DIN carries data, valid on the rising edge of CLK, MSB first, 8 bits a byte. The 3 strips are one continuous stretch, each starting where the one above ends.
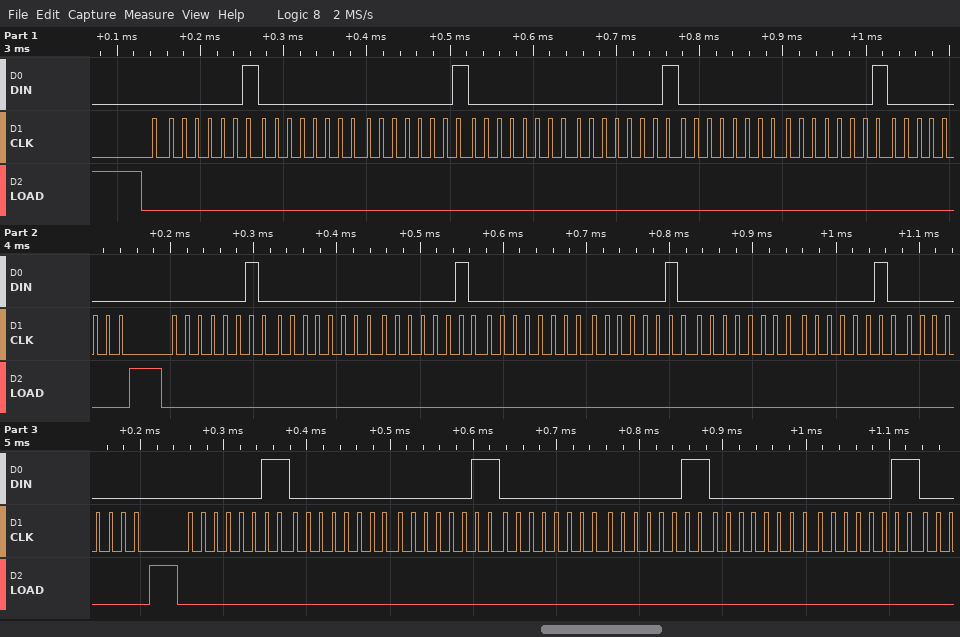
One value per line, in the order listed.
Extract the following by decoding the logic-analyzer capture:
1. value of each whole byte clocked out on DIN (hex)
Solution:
01 00 01 00 01 00 01 00 02 00 02 00 02 00 02 00 03 00 03 00 03 00 03
